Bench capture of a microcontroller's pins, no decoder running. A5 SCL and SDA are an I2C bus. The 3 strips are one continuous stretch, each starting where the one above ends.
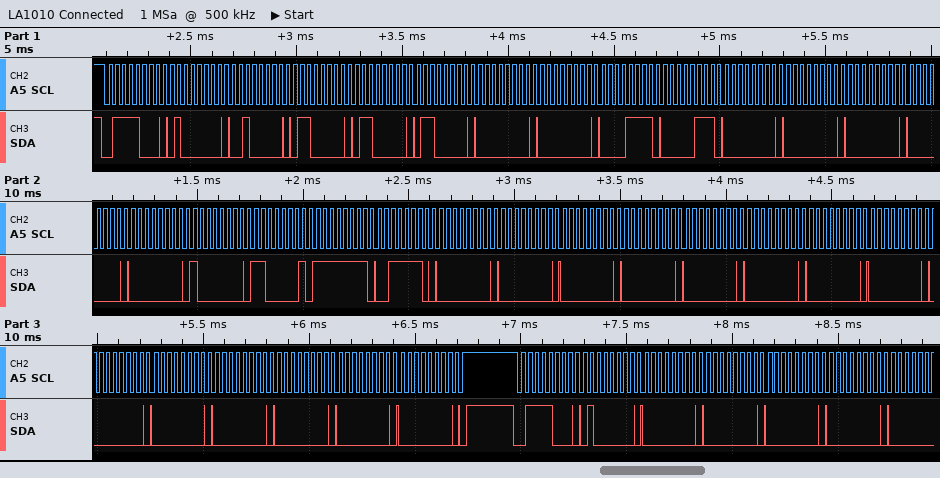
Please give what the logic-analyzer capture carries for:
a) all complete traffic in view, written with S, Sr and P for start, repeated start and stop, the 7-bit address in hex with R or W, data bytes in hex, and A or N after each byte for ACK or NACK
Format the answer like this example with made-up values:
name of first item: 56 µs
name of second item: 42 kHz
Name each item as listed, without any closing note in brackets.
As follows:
all complete traffic in view, written with S, Sr and P for start, repeated start and stop, the 7-bit address in hex with R or W, data bytes in hex, and A or N after each byte for ACK or NACK: S 3CW A 40 A 20 A 60 A 60 A 60 A 00 A 00 A 0F A 07 A 00 A 00 A 00 A 00 A 00 A 80 A C1 A FF A 3E A 00 A 00 A 00 A 00 A 00 A 00 A 00 A 00 A 00 A 00 A 00 A 00 A 00 A 00 A P S 3CW A 40 A 00 A 00 A 00 A 00 A
